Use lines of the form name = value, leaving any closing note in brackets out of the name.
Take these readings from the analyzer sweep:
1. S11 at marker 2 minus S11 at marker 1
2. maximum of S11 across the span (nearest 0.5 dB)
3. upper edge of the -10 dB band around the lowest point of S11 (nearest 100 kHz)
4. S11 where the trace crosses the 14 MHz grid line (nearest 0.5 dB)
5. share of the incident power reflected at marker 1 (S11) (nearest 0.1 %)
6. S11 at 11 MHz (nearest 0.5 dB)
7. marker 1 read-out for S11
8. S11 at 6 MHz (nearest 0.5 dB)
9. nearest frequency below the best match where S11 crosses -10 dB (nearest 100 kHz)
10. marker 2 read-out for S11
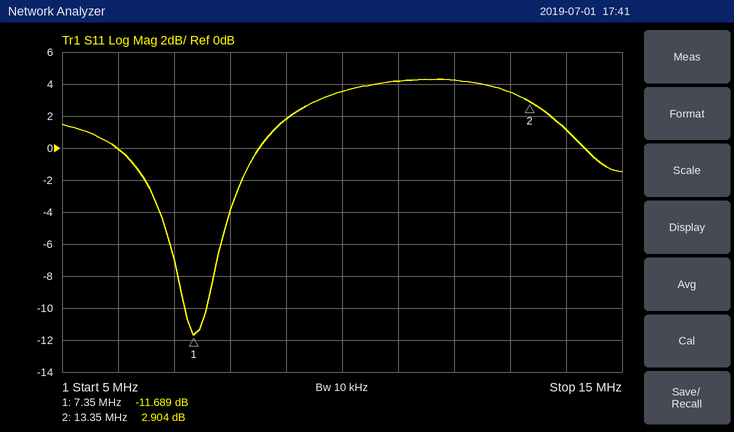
S11 at marker 2 minus S11 at marker 1 = 14.593 dB
maximum of S11 across the span = 4.5 dB
upper edge of the -10 dB band around the lowest point of S11 = 7.6 MHz
S11 where the trace crosses the 14 MHz grid line = 1.0 dB
share of the incident power reflected at marker 1 (S11) = 6.8 %
S11 at 11 MHz = 4.0 dB
marker 1 read-out for S11 = -11.689 dB
S11 at 6 MHz = 0.0 dB
nearest frequency below the best match where S11 crosses -10 dB = 7.2 MHz
marker 2 read-out for S11 = 2.904 dB
